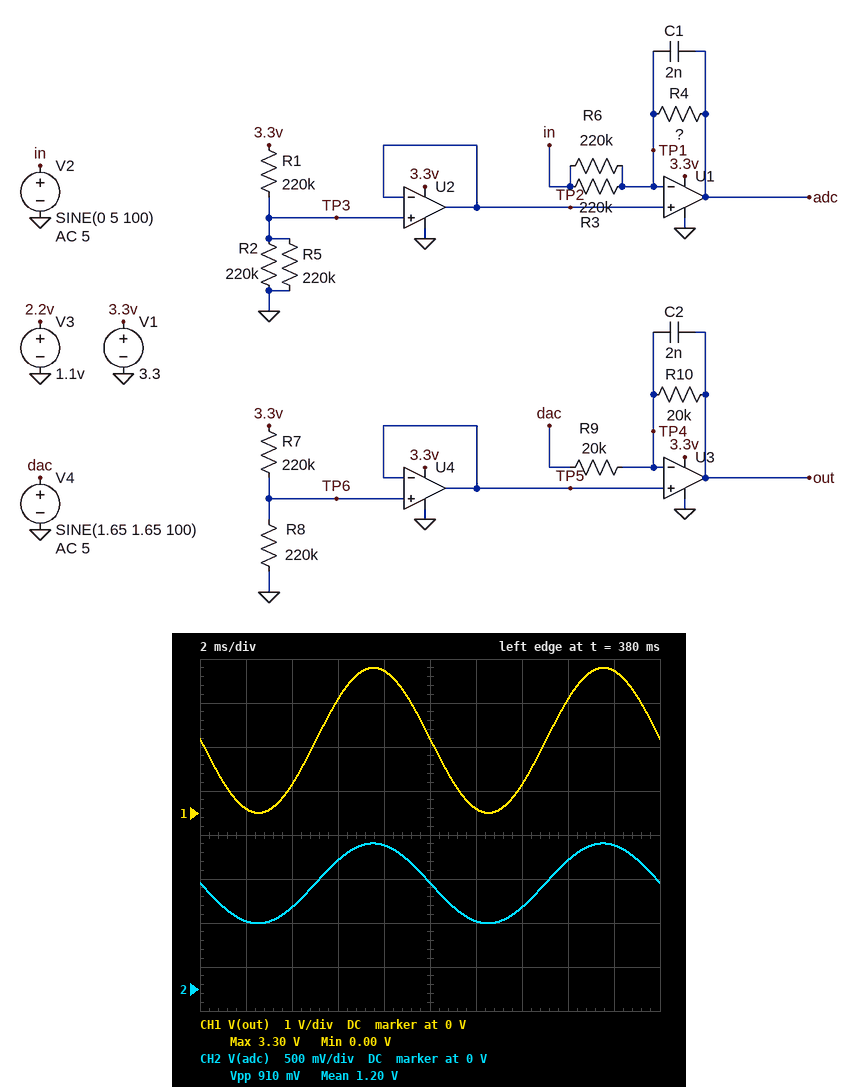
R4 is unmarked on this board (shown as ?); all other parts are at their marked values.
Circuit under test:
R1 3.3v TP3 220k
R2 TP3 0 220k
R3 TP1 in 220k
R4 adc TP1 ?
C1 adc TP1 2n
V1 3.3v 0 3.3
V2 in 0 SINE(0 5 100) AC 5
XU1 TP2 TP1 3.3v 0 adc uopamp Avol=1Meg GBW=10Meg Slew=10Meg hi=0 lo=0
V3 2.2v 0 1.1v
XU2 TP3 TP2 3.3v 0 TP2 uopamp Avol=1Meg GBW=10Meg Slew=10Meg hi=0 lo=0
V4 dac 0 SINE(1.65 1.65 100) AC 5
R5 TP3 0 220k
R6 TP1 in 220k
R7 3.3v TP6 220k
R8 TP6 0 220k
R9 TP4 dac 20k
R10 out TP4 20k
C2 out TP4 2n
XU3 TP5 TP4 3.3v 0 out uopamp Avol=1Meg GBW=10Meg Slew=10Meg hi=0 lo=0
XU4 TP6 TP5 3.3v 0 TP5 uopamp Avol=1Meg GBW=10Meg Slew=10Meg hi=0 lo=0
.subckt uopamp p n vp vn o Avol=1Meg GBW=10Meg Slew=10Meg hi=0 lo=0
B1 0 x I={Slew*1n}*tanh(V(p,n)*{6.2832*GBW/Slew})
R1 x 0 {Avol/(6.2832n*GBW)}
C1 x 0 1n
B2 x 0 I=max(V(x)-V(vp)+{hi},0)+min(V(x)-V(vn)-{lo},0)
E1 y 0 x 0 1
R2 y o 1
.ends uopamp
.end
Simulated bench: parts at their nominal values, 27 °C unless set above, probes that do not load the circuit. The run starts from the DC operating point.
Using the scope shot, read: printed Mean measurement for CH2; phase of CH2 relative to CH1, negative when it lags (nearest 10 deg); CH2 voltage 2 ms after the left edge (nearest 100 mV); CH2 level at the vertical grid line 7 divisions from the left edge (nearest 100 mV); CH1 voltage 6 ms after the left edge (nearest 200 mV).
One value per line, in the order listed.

1.20 V
0 deg
800 mV
900 mV
2.6 V
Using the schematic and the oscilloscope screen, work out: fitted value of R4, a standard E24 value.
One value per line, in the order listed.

10 kΩ
